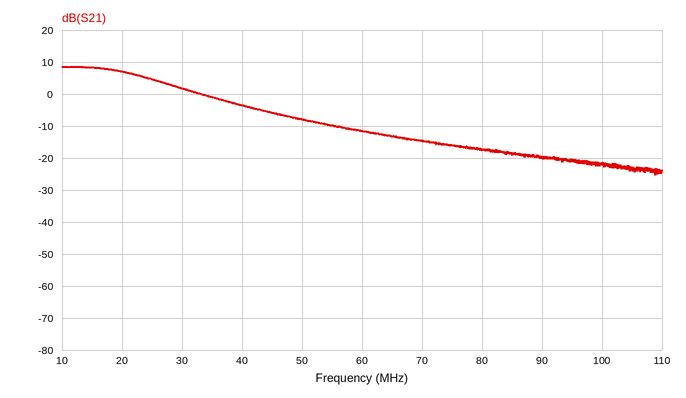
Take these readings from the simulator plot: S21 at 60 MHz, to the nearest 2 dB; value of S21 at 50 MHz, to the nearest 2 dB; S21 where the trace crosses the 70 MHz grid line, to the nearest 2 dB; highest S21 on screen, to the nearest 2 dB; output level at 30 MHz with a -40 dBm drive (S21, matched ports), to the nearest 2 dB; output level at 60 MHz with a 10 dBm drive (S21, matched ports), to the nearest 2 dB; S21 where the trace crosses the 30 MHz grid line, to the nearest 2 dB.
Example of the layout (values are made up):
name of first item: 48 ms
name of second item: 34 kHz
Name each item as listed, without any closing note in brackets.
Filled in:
S21 at 60 MHz, to the nearest 2 dB: -12 dB
value of S21 at 50 MHz, to the nearest 2 dB: -8 dB
S21 where the trace crosses the 70 MHz grid line, to the nearest 2 dB: -14 dB
highest S21 on screen, to the nearest 2 dB: 8 dB
output level at 30 MHz with a -40 dBm drive (S21, matched ports), to the nearest 2 dB: -38 dBm
output level at 60 MHz with a 10 dBm drive (S21, matched ports), to the nearest 2 dB: -2 dBm
S21 where the trace crosses the 30 MHz grid line, to the nearest 2 dB: 2 dB
